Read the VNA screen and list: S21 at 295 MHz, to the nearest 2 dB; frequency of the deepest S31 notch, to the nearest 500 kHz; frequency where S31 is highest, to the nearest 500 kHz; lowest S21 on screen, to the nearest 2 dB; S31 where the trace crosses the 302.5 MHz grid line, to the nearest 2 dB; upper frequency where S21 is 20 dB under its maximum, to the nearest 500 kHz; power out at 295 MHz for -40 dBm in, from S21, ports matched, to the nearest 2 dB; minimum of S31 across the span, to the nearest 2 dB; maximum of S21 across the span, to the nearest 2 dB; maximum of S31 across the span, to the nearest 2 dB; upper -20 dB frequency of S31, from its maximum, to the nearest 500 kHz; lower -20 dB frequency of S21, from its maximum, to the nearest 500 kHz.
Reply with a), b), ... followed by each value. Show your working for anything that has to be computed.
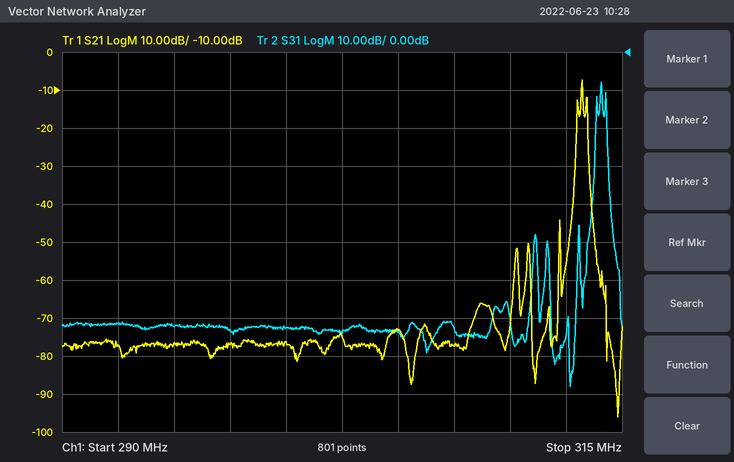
a) -76 dB
b) 312.5 MHz
c) 314.0 MHz
d) -96 dB
e) -74 dB
f) 313.5 MHz
g) -40 dBm + (-76 dB) = -116 dBm
h) -88 dB
i) -8 dB
j) -8 dB
k) 314.5 MHz
l) 313.0 MHz
